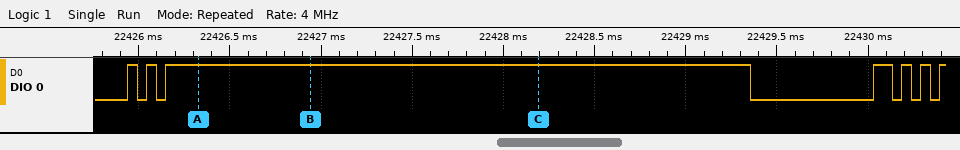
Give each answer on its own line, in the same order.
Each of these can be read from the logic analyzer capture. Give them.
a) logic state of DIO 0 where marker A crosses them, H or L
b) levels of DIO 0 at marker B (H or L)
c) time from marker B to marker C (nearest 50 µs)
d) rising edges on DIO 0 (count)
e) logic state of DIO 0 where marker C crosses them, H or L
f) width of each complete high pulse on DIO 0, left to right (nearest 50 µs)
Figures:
DIO 0=H
DIO 0=H
1250 µs
7
DIO 0=H
50 µs, 50 µs, 3200 µs, 100 µs, 50 µs, 50 µs
